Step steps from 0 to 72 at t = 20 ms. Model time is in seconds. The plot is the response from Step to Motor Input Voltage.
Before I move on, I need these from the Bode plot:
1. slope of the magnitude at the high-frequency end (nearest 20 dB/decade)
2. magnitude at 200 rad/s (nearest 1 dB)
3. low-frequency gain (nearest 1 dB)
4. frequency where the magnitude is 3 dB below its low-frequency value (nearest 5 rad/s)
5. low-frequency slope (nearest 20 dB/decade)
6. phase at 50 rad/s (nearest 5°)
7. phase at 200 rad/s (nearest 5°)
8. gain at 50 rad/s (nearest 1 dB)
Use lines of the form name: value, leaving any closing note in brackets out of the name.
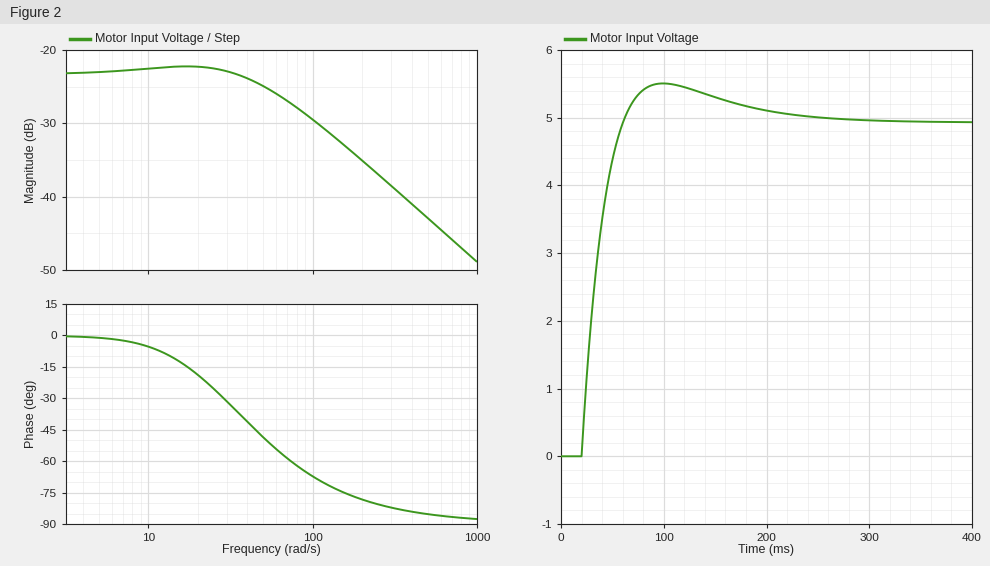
slope of the magnitude at the high-frequency end: -20 dB/decade
magnitude at 200 rad/s: -35 dB
low-frequency gain: -23 dB
frequency where the magnitude is 3 dB below its low-frequency value: 60 rad/s
low-frequency slope: 0 dB/decade
phase at 50 rad/s: -50°
phase at 200 rad/s: -80°
gain at 50 rad/s: -25 dB
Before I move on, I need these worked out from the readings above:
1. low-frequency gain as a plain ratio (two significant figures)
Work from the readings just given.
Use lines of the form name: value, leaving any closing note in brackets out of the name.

low-frequency gain as a plain ratio: 0.071
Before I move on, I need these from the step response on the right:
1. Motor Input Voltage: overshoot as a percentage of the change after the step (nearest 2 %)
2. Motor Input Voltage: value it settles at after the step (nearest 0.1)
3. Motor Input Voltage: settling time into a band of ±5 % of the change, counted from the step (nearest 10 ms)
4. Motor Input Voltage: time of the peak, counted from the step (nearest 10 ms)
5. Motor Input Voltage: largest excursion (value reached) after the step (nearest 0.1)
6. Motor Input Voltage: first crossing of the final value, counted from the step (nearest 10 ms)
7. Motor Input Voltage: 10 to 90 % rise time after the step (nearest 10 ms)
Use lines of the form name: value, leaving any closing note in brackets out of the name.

Motor Input Voltage: overshoot as a percentage of the change after the step: 12 %
Motor Input Voltage: value it settles at after the step: 4.9
Motor Input Voltage: settling time into a band of ±5 % of the change, counted from the step: 160 ms
Motor Input Voltage: time of the peak, counted from the step: 80 ms
Motor Input Voltage: largest excursion (value reached) after the step: 5.5
Motor Input Voltage: first crossing of the final value, counted from the step: 40 ms
Motor Input Voltage: 10 to 90 % rise time after the step: 30 ms
